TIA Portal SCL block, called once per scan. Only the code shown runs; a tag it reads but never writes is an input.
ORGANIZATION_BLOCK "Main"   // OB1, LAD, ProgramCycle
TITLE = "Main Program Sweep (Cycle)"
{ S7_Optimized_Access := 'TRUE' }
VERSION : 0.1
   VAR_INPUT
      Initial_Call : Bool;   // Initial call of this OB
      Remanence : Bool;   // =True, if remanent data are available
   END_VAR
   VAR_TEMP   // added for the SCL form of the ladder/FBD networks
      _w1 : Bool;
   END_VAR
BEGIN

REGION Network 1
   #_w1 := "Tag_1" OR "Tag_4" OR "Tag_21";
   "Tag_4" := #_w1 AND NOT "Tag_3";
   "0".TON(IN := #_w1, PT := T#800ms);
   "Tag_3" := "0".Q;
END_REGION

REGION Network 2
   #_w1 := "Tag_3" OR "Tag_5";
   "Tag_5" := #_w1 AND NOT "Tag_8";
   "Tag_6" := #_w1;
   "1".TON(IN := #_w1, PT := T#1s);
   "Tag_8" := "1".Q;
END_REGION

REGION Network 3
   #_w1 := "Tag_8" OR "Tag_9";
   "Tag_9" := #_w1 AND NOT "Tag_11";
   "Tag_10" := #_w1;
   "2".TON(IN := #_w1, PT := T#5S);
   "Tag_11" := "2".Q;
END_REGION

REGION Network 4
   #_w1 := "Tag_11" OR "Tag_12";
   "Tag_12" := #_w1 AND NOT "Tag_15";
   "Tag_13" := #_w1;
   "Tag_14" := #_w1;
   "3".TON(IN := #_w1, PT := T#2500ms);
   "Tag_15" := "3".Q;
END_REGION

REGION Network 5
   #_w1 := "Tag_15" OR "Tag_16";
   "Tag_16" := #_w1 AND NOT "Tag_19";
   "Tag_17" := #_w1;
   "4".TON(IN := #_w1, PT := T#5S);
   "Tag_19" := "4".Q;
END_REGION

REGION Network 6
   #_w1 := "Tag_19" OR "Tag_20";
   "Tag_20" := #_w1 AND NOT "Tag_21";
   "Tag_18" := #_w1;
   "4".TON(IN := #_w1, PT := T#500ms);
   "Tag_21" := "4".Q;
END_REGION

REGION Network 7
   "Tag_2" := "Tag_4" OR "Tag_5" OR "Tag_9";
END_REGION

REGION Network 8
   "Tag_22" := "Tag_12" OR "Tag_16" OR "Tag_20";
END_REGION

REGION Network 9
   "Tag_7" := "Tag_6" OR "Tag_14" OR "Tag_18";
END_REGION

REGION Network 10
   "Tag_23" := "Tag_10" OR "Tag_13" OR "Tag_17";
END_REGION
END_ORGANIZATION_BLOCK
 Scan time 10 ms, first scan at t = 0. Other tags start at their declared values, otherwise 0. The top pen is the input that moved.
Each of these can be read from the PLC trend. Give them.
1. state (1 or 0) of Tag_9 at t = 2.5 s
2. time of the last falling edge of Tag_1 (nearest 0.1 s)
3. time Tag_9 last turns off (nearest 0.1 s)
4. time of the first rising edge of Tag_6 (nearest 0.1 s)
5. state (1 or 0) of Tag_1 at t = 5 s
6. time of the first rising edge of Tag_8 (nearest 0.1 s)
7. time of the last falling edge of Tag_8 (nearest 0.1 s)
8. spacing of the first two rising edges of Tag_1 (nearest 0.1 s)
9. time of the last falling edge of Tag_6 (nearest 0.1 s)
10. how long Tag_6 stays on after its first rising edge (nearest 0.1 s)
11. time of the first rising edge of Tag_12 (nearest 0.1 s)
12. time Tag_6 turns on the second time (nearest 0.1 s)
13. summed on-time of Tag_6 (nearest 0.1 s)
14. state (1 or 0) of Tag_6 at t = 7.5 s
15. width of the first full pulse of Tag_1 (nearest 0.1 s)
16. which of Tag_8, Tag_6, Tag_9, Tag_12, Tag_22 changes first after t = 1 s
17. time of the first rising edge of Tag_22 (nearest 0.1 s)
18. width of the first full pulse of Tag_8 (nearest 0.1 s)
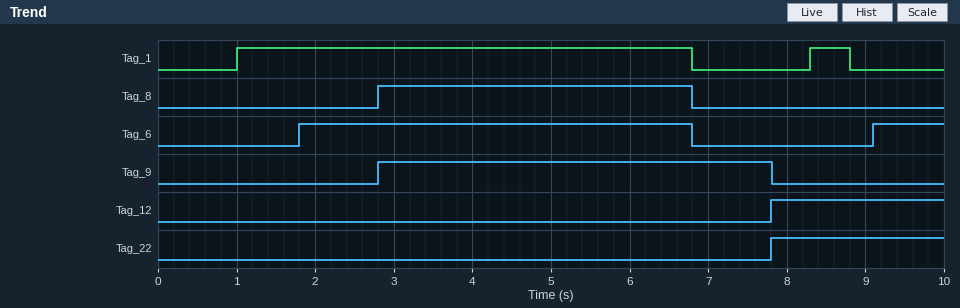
0
8.8 s
7.8 s
1.8 s
1
2.8 s
6.8 s
7.3 s
6.8 s
5.0 s
7.8 s
9.1 s
5.9 s
0
5.8 s
Tag_6
7.8 s
4.0 s
